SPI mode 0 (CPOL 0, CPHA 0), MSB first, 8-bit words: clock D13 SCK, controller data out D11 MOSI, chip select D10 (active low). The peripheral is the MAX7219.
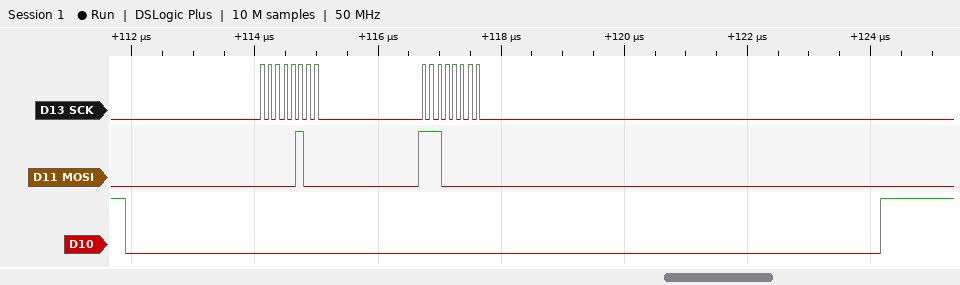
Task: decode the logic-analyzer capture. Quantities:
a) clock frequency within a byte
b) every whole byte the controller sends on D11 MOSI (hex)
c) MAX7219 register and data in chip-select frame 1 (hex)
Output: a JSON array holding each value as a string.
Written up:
["8 MHz", "04 E0", "register 0x4, data 0xE0"]
